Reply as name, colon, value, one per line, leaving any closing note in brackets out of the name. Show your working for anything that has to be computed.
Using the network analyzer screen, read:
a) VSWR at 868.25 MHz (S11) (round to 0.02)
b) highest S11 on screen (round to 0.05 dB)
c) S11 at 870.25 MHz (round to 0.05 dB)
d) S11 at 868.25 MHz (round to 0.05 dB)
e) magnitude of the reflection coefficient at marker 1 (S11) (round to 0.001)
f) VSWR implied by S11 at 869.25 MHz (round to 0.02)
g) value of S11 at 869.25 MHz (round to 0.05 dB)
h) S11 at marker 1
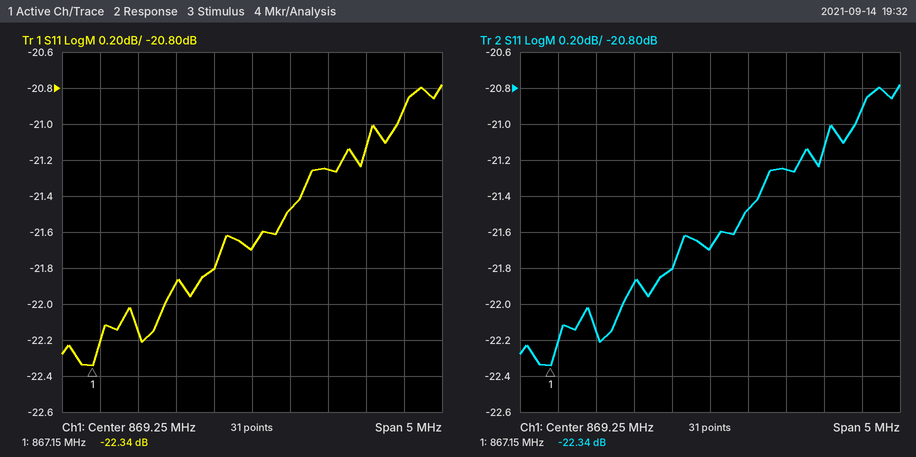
VSWR at 868.25 MHz (S11): |Γ| = 10^(-21.9/20) = 0.0804; VSWR = (1 + 0.0804)/(1 − 0.0804) ≈ 1.17, so 1.18 to the nearest 0.02
highest S11 on screen: -20.80 dB
S11 at 870.25 MHz: -21.25 dB
S11 at 868.25 MHz: -21.90 dB
magnitude of the reflection coefficient at marker 1 (S11): 10^(-22.34/20) ≈ 0.076
VSWR implied by S11 at 869.25 MHz: |Γ| = 10^(-21.7/20) = 0.0822; VSWR = (1 + 0.0822)/(1 − 0.0822) ≈ 1.18
value of S11 at 869.25 MHz: -21.70 dB
S11 at marker 1: -22.34 dB
